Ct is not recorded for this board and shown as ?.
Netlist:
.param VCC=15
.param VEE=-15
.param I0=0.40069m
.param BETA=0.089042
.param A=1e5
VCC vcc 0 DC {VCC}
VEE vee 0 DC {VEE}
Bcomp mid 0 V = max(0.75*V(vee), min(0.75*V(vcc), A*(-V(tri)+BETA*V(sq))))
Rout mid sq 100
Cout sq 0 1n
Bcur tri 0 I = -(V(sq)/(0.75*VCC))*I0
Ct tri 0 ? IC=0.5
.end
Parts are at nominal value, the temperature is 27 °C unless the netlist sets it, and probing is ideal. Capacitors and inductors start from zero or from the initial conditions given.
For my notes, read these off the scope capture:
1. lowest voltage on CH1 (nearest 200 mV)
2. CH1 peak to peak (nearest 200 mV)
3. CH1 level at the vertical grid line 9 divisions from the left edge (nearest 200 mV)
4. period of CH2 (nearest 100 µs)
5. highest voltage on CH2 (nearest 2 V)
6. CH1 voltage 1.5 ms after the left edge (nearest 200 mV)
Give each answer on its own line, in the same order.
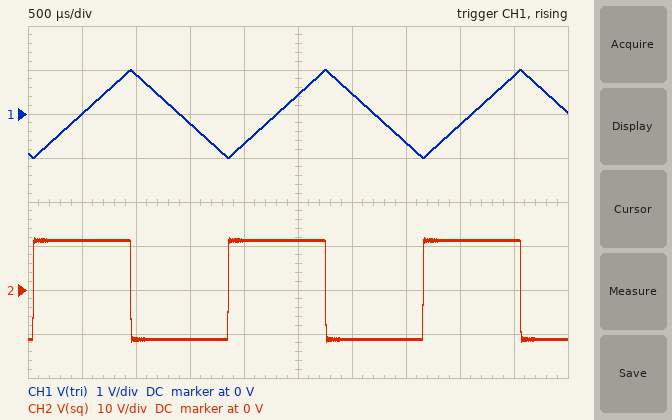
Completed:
-1.0 V
2.0 V
800 mV
1.8 ms
12 V
-200 mV
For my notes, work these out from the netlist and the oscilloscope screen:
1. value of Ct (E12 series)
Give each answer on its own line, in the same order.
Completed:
180 nF
